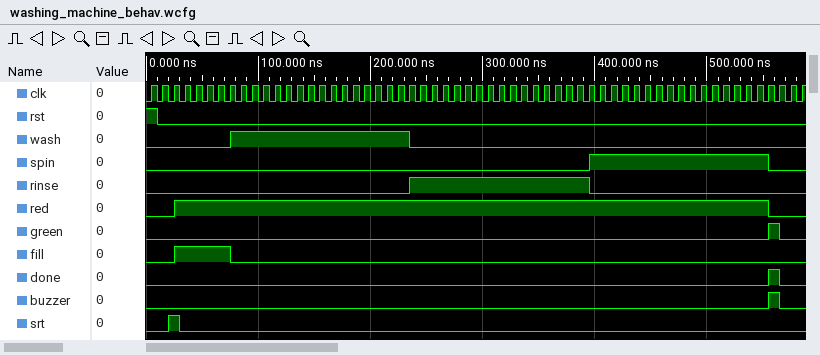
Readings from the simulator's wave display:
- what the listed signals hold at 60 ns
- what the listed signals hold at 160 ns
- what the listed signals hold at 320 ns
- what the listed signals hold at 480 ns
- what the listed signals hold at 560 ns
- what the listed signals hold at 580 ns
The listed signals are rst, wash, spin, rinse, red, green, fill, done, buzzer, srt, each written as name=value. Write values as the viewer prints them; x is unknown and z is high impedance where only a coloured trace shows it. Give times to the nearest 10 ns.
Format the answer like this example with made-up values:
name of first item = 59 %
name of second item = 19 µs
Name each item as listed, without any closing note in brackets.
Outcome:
what the listed signals hold at 60 ns = rst=0, wash=0, spin=0, rinse=0, red=1, green=0, fill=1, done=0, buzzer=0, srt=0
what the listed signals hold at 160 ns = rst=0, wash=1, spin=0, rinse=0, red=1, green=0, fill=0, done=0, buzzer=0, srt=0
what the listed signals hold at 320 ns = rst=0, wash=0, spin=0, rinse=1, red=1, green=0, fill=0, done=0, buzzer=0, srt=0
what the listed signals hold at 480 ns = rst=0, wash=0, spin=1, rinse=0, red=1, green=0, fill=0, done=0, buzzer=0, srt=0
what the listed signals hold at 560 ns = rst=0, wash=0, spin=0, rinse=0, red=0, green=1, fill=0, done=1, buzzer=1, srt=0
what the listed signals hold at 580 ns = rst=0, wash=0, spin=0, rinse=0, red=0, green=0, fill=0, done=0, buzzer=0, srt=0
